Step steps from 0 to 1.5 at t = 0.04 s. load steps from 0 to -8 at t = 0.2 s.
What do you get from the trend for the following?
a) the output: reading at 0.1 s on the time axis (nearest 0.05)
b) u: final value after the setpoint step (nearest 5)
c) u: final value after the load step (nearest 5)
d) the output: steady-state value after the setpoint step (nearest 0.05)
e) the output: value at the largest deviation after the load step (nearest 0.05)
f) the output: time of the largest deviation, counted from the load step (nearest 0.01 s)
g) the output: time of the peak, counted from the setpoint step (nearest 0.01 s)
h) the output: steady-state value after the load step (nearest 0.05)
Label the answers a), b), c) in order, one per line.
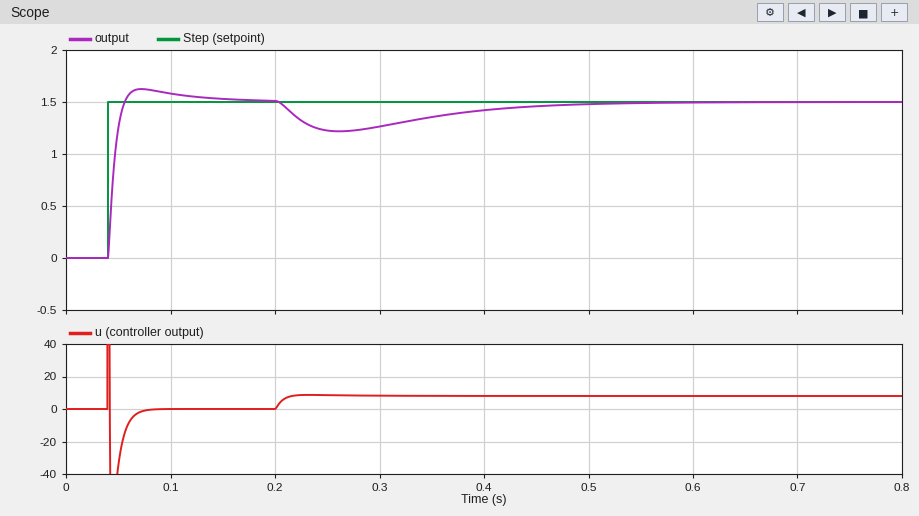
a) 1.60
b) 0
c) 10
d) 1.50
e) 1.20
f) 0.06 s
g) 0.03 s
h) 1.50
